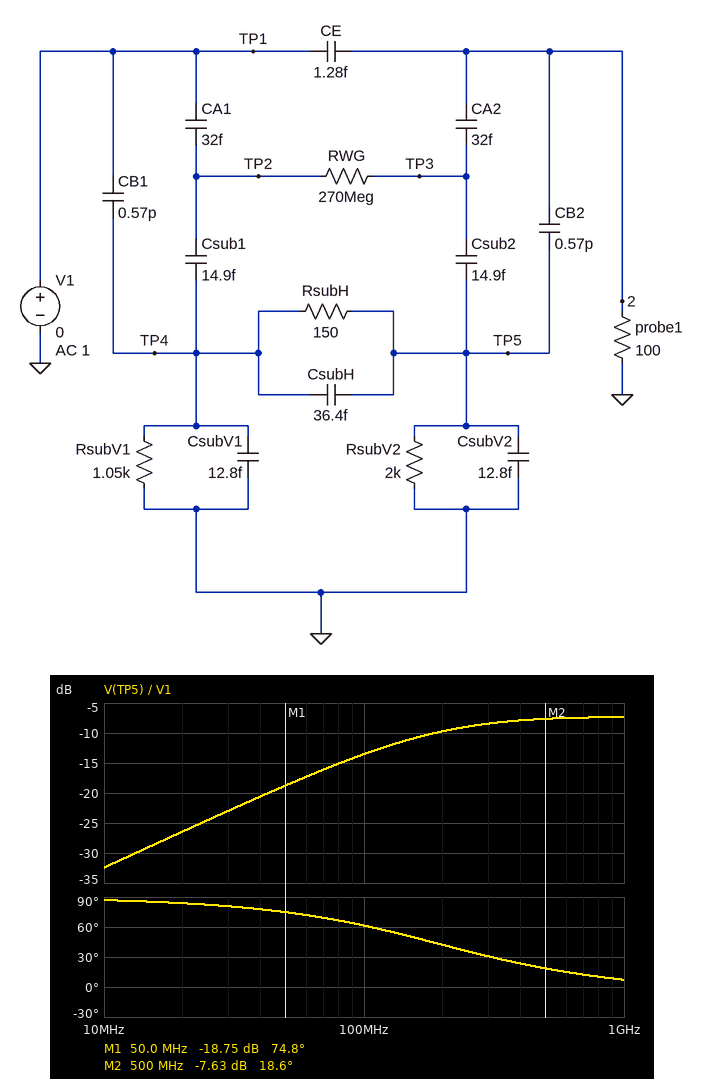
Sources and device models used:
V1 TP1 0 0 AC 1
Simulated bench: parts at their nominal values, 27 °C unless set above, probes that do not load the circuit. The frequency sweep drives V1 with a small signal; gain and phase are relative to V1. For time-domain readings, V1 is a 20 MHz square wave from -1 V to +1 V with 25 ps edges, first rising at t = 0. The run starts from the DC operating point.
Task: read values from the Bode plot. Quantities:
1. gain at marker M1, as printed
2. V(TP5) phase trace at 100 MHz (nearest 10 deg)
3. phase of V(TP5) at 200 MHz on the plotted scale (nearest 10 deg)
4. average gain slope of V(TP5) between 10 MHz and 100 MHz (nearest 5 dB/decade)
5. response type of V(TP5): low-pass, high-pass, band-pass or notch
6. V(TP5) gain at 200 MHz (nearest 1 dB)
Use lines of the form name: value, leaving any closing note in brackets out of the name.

gain at marker M1, as printed: -18.75 dB
V(TP5) phase trace at 100 MHz: 60 deg
phase of V(TP5) at 200 MHz on the plotted scale: 40 deg
average gain slope of V(TP5) between 10 MHz and 100 MHz: 20 dB/decade
response type of V(TP5): low-pass, high-pass, band-pass or notch: high-pass
V(TP5) gain at 200 MHz: -10 dB
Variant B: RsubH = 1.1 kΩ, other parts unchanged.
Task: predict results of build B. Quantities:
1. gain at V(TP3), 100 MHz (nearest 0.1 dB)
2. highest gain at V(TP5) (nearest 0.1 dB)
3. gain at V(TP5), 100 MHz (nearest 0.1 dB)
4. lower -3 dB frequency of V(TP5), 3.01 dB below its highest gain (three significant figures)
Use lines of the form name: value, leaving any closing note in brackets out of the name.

gain at V(TP3), 100 MHz: -25.9 dB
highest gain at V(TP5): -11.9 dB
gain at V(TP5), 100 MHz: -16.0 dB
lower -3 dB frequency of V(TP5), 3.01 dB below its highest gain: 120 MHz
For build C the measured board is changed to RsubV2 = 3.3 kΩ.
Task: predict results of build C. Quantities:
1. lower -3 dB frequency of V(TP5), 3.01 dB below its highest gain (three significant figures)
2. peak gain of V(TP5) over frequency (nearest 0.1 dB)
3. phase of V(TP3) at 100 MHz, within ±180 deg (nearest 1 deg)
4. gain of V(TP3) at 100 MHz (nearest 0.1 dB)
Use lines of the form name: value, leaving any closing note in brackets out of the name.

lower -3 dB frequency of V(TP5), 3.01 dB below its highest gain: 149 MHz
peak gain of V(TP5) over frequency: -7.2 dB
phase of V(TP3) at 100 MHz, within ±180 deg: 62 deg
gain of V(TP3) at 100 MHz: -22.4 dB
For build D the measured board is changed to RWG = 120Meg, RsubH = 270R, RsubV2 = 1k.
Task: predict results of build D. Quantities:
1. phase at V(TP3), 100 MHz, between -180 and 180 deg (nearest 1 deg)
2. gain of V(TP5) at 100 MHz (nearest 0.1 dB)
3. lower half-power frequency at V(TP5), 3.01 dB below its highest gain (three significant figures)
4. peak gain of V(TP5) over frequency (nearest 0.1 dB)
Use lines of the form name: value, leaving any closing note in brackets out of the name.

phase at V(TP3), 100 MHz, between -180 and 180 deg: 71 deg
gain of V(TP5) at 100 MHz: -16.3 dB
lower half-power frequency at V(TP5), 3.01 dB below its highest gain: 202 MHz
peak gain of V(TP5) over frequency: -8.8 dB
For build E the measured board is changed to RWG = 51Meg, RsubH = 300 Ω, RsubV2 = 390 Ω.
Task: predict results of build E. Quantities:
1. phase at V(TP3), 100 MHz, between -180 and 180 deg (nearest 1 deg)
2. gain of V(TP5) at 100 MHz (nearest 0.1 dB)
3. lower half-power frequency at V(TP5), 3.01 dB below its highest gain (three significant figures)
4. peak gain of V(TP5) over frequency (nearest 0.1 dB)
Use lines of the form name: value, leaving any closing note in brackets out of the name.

phase at V(TP3), 100 MHz, between -180 and 180 deg: 79 deg
gain of V(TP5) at 100 MHz: -21.6 dB
lower half-power frequency at V(TP5), 3.01 dB below its highest gain: 300 MHz
peak gain of V(TP5) over frequency: -10.7 dB
